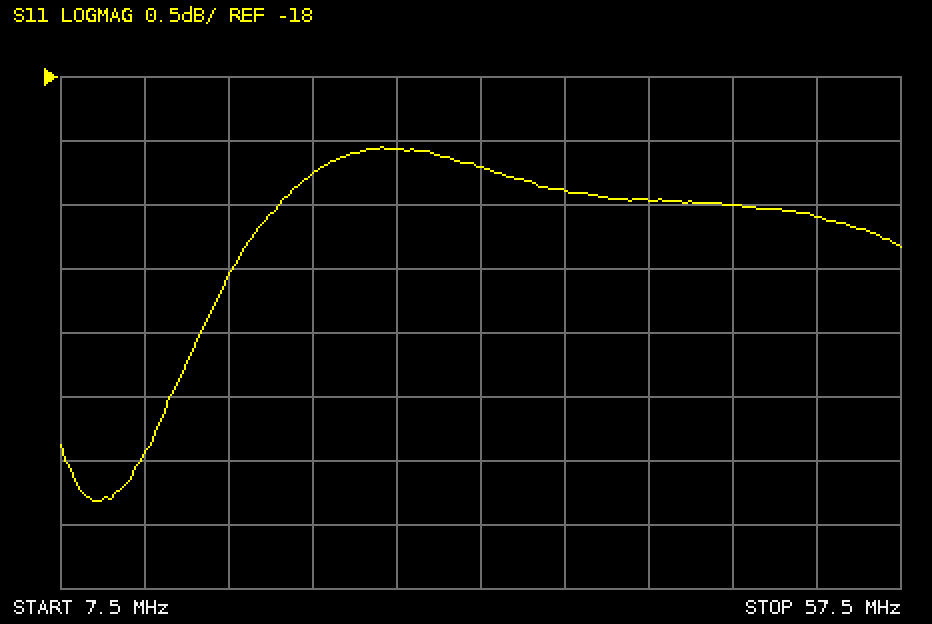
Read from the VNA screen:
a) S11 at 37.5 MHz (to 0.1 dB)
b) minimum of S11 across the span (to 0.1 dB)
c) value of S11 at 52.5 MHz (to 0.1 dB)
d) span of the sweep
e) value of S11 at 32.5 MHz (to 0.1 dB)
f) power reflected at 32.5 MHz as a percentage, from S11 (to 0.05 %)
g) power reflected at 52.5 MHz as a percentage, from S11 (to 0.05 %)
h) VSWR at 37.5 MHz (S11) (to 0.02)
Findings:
-18.9 dB
-21.3 dB
-19.1 dB
50 MHz
-18.7 dB
1.35 %
1.25 %
1.26
